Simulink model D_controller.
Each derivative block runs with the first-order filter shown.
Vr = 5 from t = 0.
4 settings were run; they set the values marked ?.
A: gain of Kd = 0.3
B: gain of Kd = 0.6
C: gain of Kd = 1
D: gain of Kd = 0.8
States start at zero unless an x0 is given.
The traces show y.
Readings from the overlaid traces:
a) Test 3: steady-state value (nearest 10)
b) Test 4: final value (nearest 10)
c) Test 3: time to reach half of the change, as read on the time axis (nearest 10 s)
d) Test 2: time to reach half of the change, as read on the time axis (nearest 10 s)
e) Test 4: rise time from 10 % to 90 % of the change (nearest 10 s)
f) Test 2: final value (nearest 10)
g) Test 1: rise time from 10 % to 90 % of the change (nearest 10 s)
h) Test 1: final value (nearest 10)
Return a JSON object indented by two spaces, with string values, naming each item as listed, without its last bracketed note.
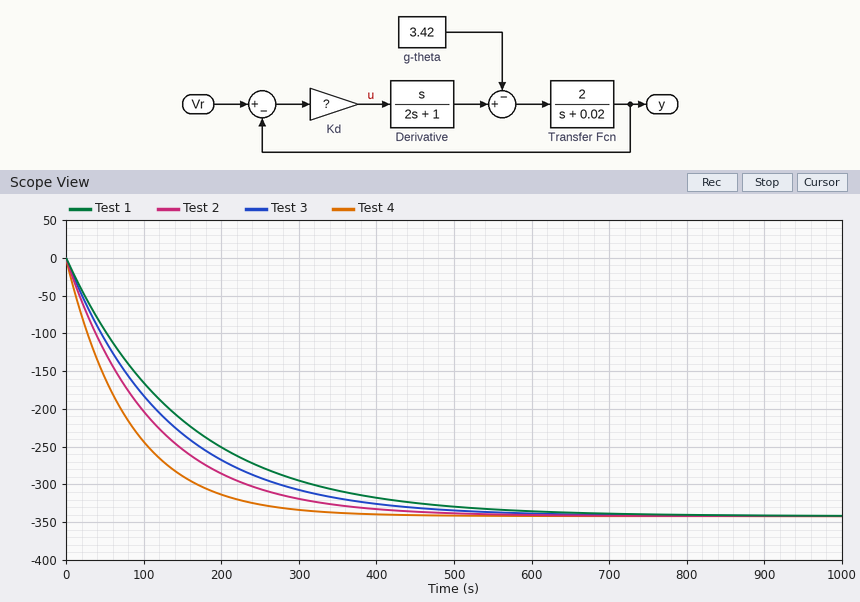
{
  "Test 3: steady-state value": "-340",
  "Test 4: final value": "-340",
  "Test 3: time to reach half of the change, as read on the time axis": "90 s",
  "Test 2: time to reach half of the change, as read on the time axis": "80 s",
  "Test 4: rise time from 10 % to 90 % of the change": "180 s",
  "Test 2: final value": "-340",
  "Test 1: rise time from 10 % to 90 % of the change": "330 s",
  "Test 1: final value": "-340"
}
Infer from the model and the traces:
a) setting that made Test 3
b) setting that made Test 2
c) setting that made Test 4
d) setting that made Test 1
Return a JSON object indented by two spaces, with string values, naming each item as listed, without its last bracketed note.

{
  "setting that made Test 3": "D",
  "setting that made Test 2": "B",
  "setting that made Test 4": "A",
  "setting that made Test 1": "C"
}
